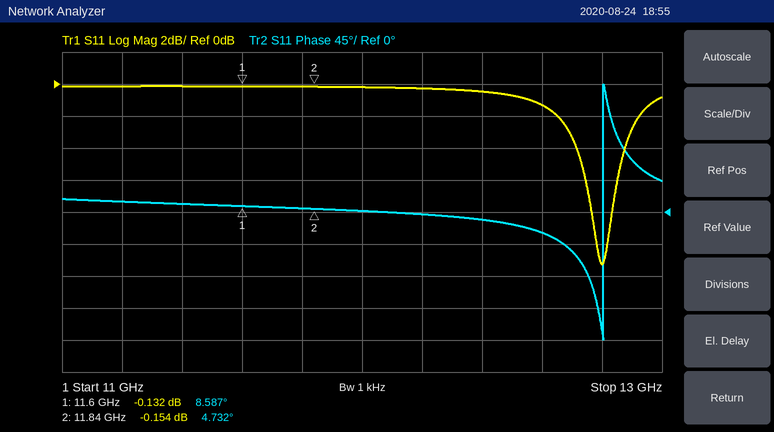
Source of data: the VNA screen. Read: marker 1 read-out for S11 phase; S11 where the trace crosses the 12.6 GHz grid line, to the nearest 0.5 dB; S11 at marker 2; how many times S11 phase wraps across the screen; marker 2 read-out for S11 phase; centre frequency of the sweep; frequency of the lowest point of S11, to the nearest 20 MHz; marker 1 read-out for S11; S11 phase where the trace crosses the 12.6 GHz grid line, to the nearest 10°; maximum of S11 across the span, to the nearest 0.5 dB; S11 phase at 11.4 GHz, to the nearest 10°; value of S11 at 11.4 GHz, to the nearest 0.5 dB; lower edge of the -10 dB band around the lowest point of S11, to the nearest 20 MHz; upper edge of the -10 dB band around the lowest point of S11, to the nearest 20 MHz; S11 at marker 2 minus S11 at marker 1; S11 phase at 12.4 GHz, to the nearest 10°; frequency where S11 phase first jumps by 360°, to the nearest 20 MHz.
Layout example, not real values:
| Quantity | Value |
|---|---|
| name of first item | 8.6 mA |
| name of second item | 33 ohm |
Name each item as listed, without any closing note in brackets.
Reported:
| Quantity | Value |
|---|---|
| marker 1 read-out for S11 phase | 8.587° |
| S11 where the trace crosses the 12.6 GHz grid line, to the nearest 0.5 dB | -1.5 dB |
| S11 at marker 2 | -0.154 dB |
| how many times S11 phase wraps across the screen | 1 |
| marker 2 read-out for S11 phase | 4.732° |
| centre frequency of the sweep | 12 GHz |
| frequency of the lowest point of S11, to the nearest 20 MHz | 12.80 GHz |
| marker 1 read-out for S11 | -0.132 dB |
| S11 phase where the trace crosses the 12.6 GHz grid line, to the nearest 10° | -30° |
| maximum of S11 across the span, to the nearest 0.5 dB | 0.0 dB |
| S11 phase at 11.4 GHz, to the nearest 10° | 10° |
| value of S11 at 11.4 GHz, to the nearest 0.5 dB | 0.0 dB |
| lower edge of the -10 dB band around the lowest point of S11, to the nearest 20 MHz | 12.78 GHz |
| upper edge of the -10 dB band around the lowest point of S11, to the nearest 20 MHz | 12.82 GHz |
| S11 at marker 2 minus S11 at marker 1 | -0.022 dB |
| S11 phase at 12.4 GHz, to the nearest 10° | -10° |
| frequency where S11 phase first jumps by 360°, to the nearest 20 MHz | 12.80 GHz |
